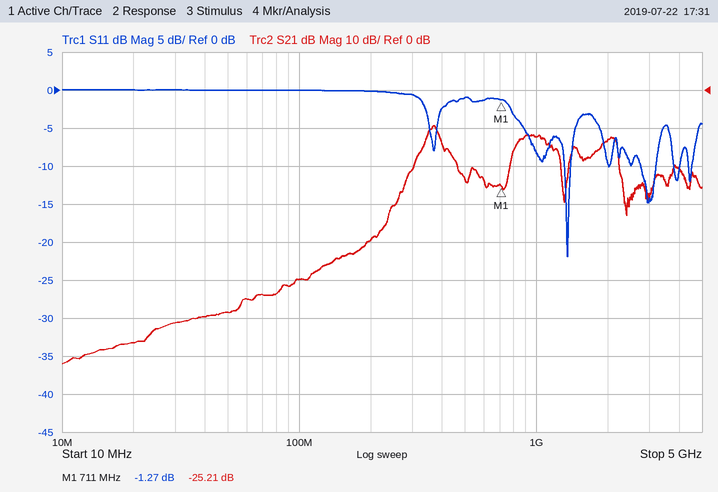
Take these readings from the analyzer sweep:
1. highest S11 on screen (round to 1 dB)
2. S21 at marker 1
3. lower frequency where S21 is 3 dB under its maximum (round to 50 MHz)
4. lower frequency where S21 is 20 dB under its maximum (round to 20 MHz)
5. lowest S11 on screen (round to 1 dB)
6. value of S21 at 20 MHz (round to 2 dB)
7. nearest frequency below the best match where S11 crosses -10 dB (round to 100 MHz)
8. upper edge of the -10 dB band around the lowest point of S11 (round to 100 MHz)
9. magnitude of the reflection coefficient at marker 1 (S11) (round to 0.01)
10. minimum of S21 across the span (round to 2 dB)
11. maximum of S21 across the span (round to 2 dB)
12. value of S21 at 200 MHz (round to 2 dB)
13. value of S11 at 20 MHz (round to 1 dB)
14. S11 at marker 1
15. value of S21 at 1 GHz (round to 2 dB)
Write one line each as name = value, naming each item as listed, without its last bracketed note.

highest S11 on screen = 0 dB
S21 at marker 1 = -25.21 dB
lower frequency where S21 is 3 dB under its maximum = 350 MHz
lower frequency where S21 is 20 dB under its maximum = 260 MHz
lowest S11 on screen = -22 dB
value of S21 at 20 MHz = -66 dB
nearest frequency below the best match where S11 crosses -10 dB = 1.3 GHz
upper edge of the -10 dB band around the lowest point of S11 = 1.4 GHz
magnitude of the reflection coefficient at marker 1 (S11) = 0.86
minimum of S21 across the span = -72 dB
maximum of S21 across the span = -10 dB
value of S21 at 200 MHz = -40 dB
value of S11 at 20 MHz = 0 dB
S11 at marker 1 = -1.27 dB
value of S21 at 1 GHz = -12 dB
